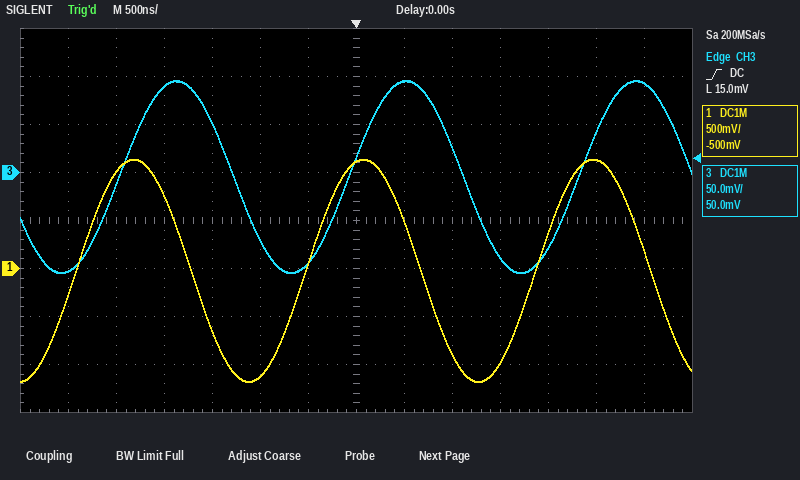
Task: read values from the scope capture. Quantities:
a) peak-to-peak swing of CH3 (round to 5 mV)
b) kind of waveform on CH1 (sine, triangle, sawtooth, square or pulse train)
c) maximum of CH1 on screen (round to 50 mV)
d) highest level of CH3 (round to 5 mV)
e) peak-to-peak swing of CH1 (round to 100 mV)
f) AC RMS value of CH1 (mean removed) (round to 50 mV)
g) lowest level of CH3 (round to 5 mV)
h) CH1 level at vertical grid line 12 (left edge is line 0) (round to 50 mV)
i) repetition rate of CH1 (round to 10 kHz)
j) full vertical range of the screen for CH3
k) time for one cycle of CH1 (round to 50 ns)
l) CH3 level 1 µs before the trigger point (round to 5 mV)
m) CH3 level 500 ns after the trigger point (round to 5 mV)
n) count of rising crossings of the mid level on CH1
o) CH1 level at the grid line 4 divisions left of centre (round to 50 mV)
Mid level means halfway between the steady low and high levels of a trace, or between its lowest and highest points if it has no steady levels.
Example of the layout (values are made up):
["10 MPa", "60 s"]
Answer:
["200 mV", "sine", "1.15 V", "95 mV", "2.30 V", "800 mV", "-105 mV", "1.15 V", "420 kHz", "400 mV", "2.40 µs", "-70 mV", "95 mV", "3", "750 mV"]
